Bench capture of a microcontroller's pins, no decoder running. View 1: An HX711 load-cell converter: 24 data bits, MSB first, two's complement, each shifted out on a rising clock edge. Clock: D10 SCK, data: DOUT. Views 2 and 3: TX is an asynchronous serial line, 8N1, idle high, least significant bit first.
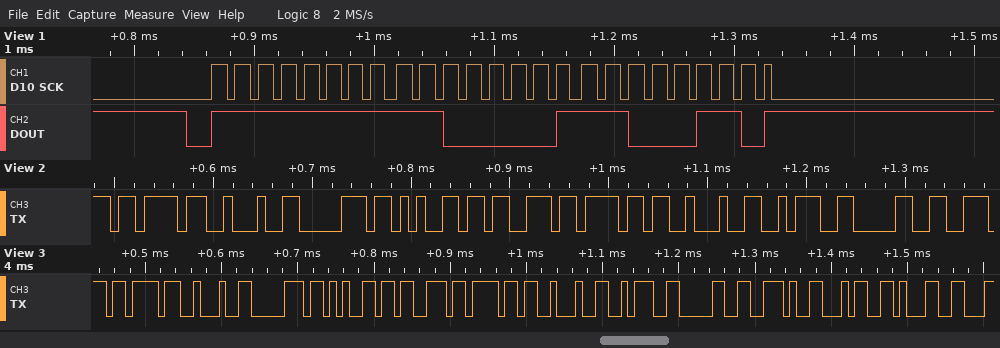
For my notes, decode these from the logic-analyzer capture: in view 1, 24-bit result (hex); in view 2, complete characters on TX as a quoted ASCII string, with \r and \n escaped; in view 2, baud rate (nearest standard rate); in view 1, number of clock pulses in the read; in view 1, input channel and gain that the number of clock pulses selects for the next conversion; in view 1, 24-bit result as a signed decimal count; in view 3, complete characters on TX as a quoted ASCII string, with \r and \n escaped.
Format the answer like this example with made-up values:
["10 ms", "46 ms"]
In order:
["0xFFC1C6", "\"{\\\"peso\\\":0\"", "115200 baud", "25", "channel A, gain 128", "-15930", "\"{\\\"peso\\\":0.41\""]
